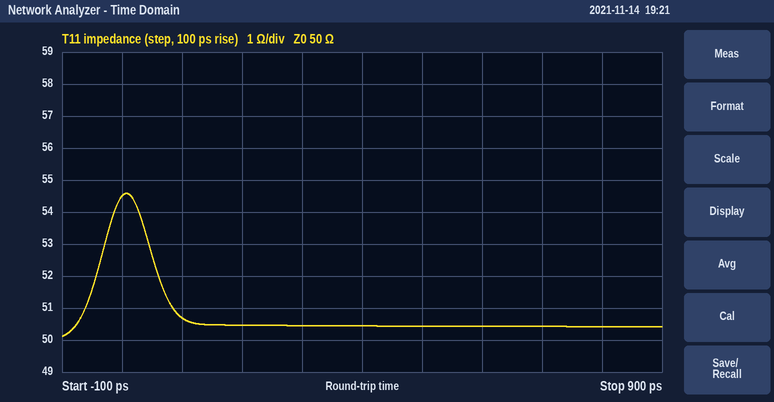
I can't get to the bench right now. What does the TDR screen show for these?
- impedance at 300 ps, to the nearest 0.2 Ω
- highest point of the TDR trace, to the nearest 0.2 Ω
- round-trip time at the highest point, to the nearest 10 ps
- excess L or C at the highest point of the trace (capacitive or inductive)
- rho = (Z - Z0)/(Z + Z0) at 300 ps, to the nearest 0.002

50.4 Ω
54.6 Ω
10 ps
inductive
+0.004
